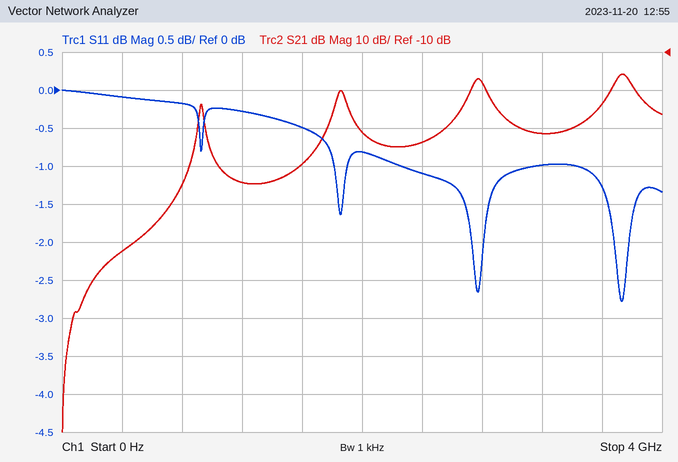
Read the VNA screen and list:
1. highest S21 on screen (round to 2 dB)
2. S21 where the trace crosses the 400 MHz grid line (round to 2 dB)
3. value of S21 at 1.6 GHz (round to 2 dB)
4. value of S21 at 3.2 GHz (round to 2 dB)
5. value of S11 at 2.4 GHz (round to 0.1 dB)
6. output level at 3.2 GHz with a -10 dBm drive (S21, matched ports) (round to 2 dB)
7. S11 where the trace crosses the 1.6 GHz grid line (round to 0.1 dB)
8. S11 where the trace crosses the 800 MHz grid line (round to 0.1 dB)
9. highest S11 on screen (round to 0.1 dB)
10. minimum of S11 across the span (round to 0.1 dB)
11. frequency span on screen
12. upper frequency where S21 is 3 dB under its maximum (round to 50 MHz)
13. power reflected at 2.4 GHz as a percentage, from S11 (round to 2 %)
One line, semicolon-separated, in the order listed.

-16 dB; -62 dB; -40 dB; -32 dB; -1.1 dB; -42 dBm; -0.5 dB; -0.2 dB; 0.0 dB; -2.8 dB; 4 GHz; 3.80 GHz; 78 %
